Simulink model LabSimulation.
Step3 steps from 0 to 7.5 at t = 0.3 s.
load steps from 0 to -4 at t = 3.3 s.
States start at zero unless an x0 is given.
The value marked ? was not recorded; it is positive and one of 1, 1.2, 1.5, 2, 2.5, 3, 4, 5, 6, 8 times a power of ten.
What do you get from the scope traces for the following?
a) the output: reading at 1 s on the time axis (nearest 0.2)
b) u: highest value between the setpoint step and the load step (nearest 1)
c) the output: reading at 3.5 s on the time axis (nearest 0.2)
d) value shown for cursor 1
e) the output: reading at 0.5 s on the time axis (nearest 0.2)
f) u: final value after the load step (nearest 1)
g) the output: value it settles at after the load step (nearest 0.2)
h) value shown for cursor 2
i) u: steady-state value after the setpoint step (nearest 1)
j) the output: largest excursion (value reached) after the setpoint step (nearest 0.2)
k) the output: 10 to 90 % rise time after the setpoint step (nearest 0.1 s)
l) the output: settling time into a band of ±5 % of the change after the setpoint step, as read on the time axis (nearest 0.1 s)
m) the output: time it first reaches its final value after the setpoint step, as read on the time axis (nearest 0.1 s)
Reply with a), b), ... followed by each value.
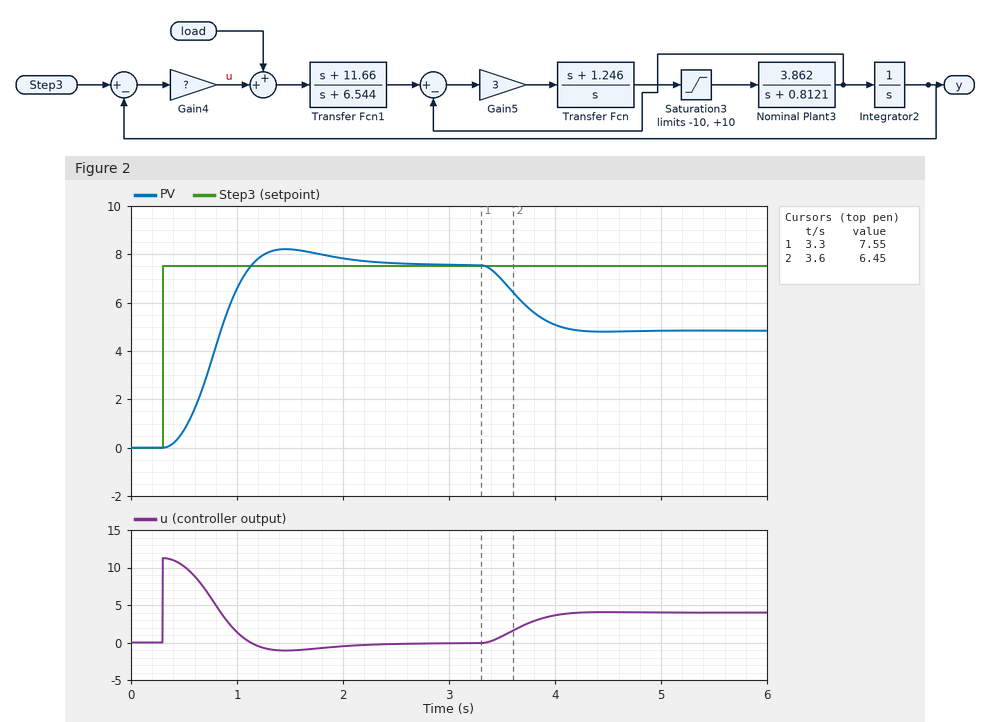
a) 6.6
b) 11
c) 7.0
d) 7.55
e) 0.8
f) 4
g) 4.8
h) 6.45
i) 0
j) 8.2
k) 0.5 s
l) 1.9 s
m) 1.1 s
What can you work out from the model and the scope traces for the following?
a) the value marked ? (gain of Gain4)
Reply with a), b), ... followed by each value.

a) 1.5
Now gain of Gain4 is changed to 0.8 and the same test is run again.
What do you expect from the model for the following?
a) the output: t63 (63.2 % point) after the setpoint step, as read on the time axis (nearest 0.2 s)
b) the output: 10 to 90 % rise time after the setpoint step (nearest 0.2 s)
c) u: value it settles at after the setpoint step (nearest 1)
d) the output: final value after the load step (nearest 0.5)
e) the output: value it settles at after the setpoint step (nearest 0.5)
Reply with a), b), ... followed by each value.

a) 1.0 s
b) 1.2 s
c) 0
d) 2.5
e) 7.5
